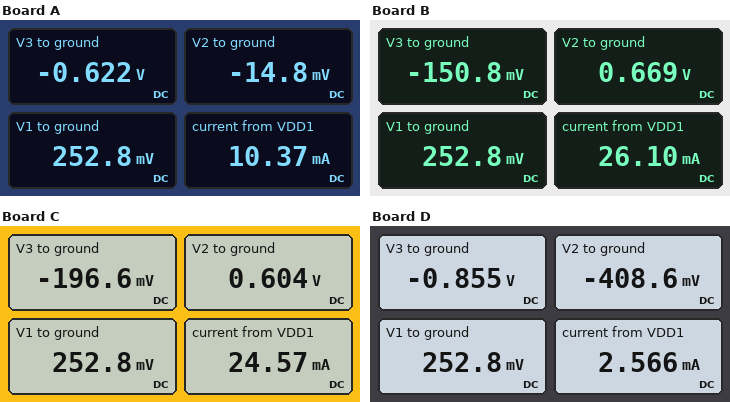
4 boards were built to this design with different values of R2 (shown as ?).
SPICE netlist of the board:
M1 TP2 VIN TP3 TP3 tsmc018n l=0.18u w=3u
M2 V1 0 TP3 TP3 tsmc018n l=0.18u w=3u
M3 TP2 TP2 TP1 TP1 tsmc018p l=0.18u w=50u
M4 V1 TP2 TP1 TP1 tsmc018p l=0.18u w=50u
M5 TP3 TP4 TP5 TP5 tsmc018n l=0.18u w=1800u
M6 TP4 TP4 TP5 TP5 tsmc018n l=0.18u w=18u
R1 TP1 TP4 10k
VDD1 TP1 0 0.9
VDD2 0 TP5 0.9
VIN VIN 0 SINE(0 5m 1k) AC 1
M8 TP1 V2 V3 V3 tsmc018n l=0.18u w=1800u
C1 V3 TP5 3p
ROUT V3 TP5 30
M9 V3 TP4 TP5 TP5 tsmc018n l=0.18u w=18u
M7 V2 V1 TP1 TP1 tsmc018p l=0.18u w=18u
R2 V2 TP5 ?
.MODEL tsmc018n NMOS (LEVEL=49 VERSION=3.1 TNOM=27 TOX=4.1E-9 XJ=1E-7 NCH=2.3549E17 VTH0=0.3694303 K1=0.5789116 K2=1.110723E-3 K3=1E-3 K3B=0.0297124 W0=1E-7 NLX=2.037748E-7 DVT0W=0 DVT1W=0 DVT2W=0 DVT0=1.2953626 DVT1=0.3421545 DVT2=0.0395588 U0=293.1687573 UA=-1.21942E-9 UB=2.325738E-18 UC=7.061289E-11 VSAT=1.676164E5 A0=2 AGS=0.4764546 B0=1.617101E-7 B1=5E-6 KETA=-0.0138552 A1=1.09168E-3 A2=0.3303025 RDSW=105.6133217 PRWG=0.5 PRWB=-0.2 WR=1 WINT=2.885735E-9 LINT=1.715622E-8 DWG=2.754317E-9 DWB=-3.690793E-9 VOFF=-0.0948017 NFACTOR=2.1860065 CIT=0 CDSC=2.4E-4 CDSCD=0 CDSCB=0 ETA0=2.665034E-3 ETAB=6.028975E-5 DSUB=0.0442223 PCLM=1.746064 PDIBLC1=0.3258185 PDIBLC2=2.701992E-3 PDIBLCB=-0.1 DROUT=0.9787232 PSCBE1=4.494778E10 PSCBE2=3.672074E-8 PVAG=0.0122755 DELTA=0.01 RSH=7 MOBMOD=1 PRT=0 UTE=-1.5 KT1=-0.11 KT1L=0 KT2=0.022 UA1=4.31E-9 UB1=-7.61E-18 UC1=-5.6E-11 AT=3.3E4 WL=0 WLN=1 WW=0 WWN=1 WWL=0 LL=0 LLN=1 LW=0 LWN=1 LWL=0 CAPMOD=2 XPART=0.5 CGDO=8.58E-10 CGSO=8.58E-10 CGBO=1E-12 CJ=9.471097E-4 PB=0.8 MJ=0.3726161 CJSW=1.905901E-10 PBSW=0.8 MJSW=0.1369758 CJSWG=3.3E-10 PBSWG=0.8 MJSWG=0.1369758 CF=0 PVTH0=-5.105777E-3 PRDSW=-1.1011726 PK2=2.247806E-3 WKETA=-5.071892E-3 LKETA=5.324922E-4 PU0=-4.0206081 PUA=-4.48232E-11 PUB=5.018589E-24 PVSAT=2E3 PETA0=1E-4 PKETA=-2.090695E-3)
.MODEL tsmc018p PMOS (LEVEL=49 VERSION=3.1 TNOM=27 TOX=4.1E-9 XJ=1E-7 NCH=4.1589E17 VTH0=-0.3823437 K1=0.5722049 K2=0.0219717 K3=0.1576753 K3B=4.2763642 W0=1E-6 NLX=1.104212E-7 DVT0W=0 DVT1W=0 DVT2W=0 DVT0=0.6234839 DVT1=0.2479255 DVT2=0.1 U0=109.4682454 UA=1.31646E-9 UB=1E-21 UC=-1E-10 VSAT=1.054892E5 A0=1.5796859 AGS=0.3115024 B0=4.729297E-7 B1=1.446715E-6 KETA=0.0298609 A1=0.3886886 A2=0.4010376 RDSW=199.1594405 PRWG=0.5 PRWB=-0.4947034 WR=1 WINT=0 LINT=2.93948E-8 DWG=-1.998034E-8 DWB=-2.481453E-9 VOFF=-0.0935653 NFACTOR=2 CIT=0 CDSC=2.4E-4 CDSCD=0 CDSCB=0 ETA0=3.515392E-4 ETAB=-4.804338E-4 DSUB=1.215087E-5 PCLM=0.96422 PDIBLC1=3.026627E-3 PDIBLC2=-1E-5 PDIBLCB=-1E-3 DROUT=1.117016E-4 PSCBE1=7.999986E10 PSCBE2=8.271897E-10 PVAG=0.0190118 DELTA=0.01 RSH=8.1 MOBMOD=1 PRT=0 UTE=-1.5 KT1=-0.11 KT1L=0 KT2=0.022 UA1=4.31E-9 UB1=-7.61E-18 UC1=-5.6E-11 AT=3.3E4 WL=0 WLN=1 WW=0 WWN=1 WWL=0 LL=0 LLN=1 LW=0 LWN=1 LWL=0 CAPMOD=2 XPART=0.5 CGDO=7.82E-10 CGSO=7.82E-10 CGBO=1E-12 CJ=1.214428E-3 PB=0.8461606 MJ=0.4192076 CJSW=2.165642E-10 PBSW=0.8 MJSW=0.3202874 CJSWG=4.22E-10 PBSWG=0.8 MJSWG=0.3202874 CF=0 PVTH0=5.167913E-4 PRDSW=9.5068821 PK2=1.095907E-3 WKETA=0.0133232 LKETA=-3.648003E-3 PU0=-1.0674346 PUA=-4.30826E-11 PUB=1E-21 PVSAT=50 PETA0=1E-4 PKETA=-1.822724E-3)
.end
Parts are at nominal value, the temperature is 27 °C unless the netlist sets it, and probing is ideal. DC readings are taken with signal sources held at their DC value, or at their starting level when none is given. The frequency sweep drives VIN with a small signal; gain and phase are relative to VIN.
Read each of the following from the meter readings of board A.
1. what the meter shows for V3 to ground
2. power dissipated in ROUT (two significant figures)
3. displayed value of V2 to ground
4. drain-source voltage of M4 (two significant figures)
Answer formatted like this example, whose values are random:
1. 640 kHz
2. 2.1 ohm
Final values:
1. -0.622 V
2. 2.6 mW
3. -14.8 mV
4. -650 mV
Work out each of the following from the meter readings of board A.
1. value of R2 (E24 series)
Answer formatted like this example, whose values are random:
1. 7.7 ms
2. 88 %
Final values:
1. 6.2 kΩ
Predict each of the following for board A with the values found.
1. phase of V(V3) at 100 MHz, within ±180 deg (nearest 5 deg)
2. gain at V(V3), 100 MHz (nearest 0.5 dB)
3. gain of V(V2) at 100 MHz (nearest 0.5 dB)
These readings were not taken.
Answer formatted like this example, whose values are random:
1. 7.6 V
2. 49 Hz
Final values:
1. 55 deg
2. 15.0 dB
3. 18.5 dB
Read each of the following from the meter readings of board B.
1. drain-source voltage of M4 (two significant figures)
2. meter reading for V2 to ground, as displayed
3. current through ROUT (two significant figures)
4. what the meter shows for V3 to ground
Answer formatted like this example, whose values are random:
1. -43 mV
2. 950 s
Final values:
1. -650 mV
2. 0.669 V
3. 25 mA
4. -150.8 mV
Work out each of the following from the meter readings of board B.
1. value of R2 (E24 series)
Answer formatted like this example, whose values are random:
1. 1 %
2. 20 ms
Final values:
1. 13 kΩ
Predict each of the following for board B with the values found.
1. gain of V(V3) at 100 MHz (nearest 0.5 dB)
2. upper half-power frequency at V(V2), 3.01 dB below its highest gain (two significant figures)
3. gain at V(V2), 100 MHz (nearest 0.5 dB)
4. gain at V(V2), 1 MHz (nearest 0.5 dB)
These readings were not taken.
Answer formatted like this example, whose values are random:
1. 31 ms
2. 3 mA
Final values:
1. 14.5 dB
2. 11 MHz
3. 17.5 dB
4. 39.0 dB
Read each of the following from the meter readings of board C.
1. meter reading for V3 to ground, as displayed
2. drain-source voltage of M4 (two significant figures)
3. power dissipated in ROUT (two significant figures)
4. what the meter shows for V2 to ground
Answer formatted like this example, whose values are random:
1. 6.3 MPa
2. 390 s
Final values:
1. -196.6 mV
2. -650 mV
3. 16 mW
4. 0.604 V
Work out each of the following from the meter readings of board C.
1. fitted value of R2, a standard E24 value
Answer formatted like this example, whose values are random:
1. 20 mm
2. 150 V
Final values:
1. 12 kΩ
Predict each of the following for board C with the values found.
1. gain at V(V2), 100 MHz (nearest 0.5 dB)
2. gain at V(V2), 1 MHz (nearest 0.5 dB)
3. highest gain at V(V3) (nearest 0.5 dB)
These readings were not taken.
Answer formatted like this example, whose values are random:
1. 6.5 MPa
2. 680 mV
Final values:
1. 18.0 dB
2. 40.5 dB
3. 37.5 dB
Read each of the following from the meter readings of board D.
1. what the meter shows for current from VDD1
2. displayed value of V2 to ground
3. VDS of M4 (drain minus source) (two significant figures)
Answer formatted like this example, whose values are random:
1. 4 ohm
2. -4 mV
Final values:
1. 2.566 mA
2. -408.6 mV
3. -650 mV
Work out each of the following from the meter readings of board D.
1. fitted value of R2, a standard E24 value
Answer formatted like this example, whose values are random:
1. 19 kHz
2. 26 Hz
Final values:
1. 3.3 kΩ
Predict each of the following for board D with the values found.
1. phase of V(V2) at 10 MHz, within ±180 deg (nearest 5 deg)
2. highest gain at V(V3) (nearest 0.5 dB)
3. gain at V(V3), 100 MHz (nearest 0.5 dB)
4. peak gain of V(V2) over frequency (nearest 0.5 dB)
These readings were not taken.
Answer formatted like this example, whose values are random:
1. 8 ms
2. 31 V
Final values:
1. 145 deg
2. 28.0 dB
3. 10.0 dB
4. 35.0 dB
